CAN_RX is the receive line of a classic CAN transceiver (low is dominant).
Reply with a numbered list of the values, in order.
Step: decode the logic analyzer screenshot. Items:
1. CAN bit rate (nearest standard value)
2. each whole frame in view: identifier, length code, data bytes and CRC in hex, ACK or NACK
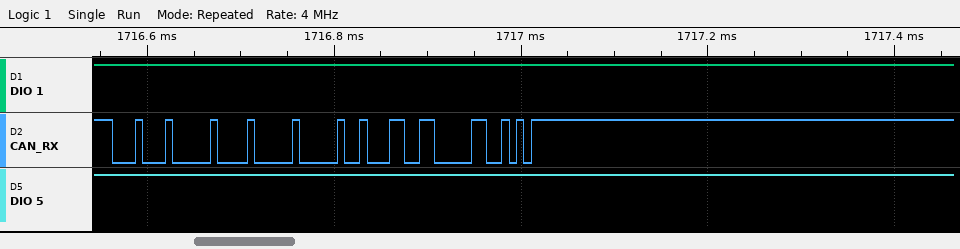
1. 125 kbit/s
2. ID 110, DLC 2, data 00 11, CRC 4C12, ACK
